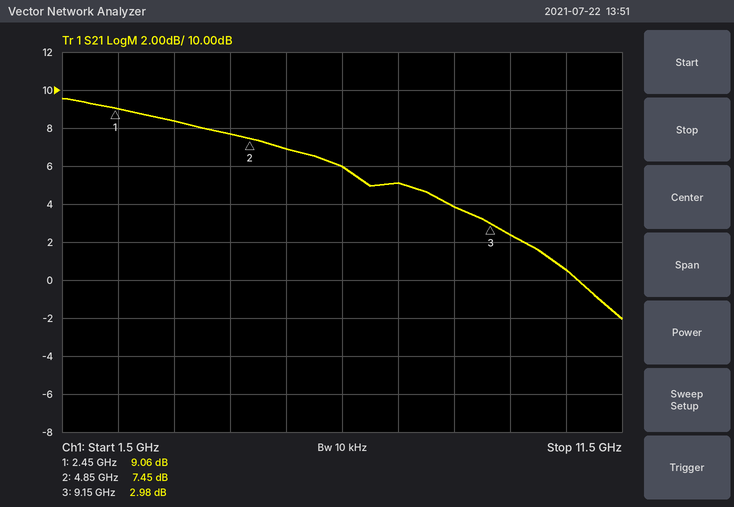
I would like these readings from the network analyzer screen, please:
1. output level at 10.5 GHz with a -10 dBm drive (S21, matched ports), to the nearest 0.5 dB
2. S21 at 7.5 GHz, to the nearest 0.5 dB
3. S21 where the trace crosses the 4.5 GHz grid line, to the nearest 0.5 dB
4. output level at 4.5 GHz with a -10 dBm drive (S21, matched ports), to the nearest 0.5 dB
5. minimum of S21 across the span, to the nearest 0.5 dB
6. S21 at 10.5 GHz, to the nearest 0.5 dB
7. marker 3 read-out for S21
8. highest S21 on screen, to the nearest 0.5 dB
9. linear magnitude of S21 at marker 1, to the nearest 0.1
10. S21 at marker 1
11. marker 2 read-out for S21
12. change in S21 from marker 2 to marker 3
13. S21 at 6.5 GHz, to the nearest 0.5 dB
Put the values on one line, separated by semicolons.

-9.5 dBm; 5.0 dB; 7.5 dB; -2.5 dBm; -2.0 dB; 0.5 dB; 2.98 dB; 9.5 dB; 2.8; 9.06 dB; 7.45 dB; -4.47 dB; 6.0 dB
